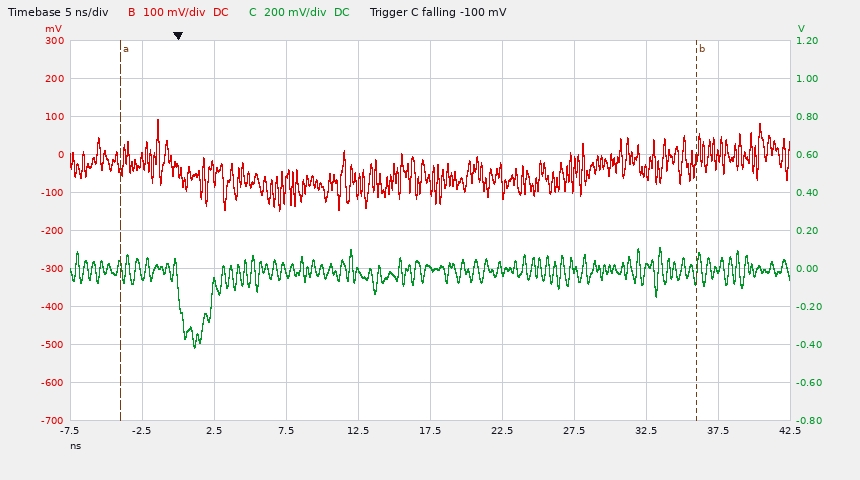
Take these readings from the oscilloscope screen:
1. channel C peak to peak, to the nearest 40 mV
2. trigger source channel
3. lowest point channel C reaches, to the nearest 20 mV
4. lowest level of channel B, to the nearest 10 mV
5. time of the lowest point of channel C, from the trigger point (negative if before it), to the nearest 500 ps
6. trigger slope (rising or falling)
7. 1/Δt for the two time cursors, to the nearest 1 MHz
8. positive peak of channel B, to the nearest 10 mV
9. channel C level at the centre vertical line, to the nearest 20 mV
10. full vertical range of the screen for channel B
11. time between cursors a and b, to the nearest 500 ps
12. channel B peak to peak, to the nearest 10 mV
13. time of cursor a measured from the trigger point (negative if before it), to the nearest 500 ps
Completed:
520 mV
channel C
-420 mV
-150 mV
+1.0 ns
falling
25 MHz
90 mV
0 mV
1 V
40.0 ns
240 mV
-4.0 ns
